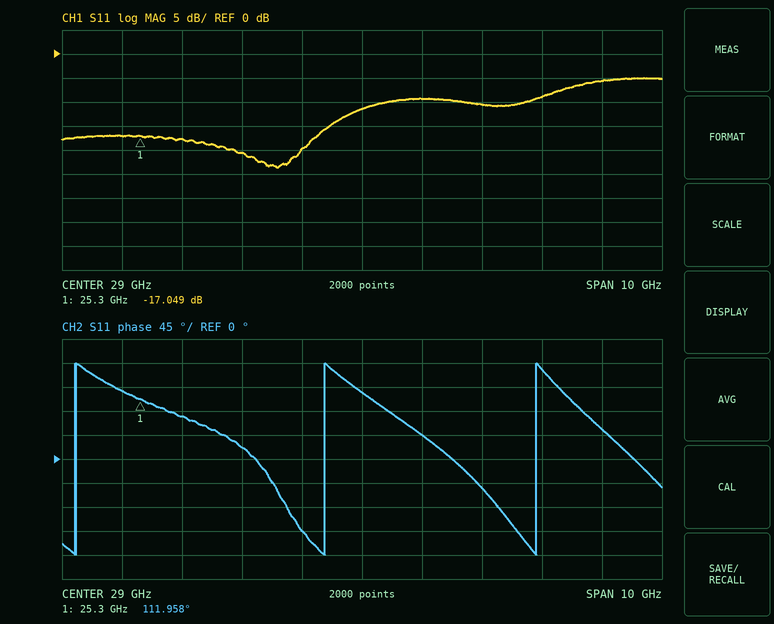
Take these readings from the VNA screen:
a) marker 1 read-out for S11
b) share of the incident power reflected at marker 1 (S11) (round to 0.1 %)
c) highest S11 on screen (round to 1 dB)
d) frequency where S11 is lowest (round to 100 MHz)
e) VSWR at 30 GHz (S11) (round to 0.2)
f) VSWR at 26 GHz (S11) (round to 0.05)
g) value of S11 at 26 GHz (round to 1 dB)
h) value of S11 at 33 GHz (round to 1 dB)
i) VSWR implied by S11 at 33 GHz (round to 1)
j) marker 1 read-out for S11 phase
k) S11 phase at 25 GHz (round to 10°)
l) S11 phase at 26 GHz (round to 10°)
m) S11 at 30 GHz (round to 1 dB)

-17.049 dB
2.0 %
-5 dB
27.6 GHz
2.0
1.30
-18 dB
-6 dB
3
111.958°
130°
80°
-9 dB
